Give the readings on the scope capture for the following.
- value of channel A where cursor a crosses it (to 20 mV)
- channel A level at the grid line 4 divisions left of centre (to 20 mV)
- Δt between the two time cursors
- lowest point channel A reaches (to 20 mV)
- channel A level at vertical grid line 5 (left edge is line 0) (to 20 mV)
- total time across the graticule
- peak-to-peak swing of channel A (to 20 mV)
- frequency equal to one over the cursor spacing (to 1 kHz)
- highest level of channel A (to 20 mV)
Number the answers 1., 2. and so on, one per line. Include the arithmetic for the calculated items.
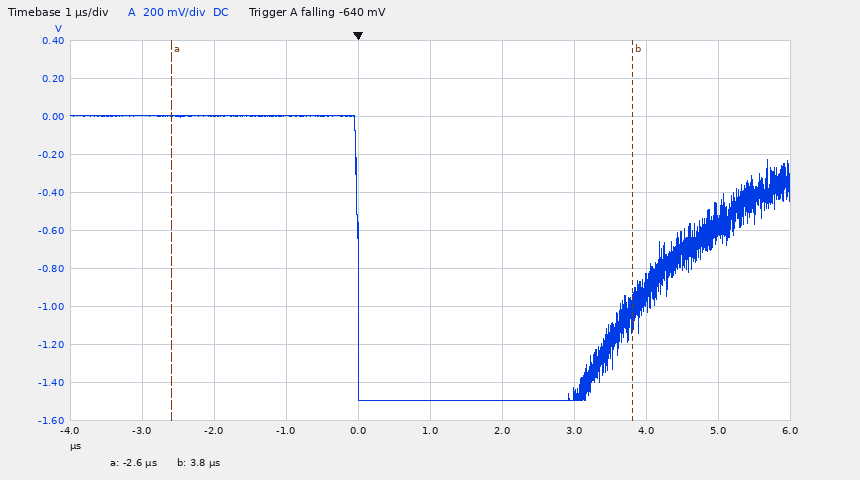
1. 0 mV
2. 0 mV
3. 3.8 µs − (-2.6 µs) = 6.4 µs
4. -1.50 V
5. -1.50 V
6. 10 µs
7. 0 mV − (-1.50 V) = 1.50 V
8. 1 / 6.4 µs ≈ 156 kHz
9. 0 mV
